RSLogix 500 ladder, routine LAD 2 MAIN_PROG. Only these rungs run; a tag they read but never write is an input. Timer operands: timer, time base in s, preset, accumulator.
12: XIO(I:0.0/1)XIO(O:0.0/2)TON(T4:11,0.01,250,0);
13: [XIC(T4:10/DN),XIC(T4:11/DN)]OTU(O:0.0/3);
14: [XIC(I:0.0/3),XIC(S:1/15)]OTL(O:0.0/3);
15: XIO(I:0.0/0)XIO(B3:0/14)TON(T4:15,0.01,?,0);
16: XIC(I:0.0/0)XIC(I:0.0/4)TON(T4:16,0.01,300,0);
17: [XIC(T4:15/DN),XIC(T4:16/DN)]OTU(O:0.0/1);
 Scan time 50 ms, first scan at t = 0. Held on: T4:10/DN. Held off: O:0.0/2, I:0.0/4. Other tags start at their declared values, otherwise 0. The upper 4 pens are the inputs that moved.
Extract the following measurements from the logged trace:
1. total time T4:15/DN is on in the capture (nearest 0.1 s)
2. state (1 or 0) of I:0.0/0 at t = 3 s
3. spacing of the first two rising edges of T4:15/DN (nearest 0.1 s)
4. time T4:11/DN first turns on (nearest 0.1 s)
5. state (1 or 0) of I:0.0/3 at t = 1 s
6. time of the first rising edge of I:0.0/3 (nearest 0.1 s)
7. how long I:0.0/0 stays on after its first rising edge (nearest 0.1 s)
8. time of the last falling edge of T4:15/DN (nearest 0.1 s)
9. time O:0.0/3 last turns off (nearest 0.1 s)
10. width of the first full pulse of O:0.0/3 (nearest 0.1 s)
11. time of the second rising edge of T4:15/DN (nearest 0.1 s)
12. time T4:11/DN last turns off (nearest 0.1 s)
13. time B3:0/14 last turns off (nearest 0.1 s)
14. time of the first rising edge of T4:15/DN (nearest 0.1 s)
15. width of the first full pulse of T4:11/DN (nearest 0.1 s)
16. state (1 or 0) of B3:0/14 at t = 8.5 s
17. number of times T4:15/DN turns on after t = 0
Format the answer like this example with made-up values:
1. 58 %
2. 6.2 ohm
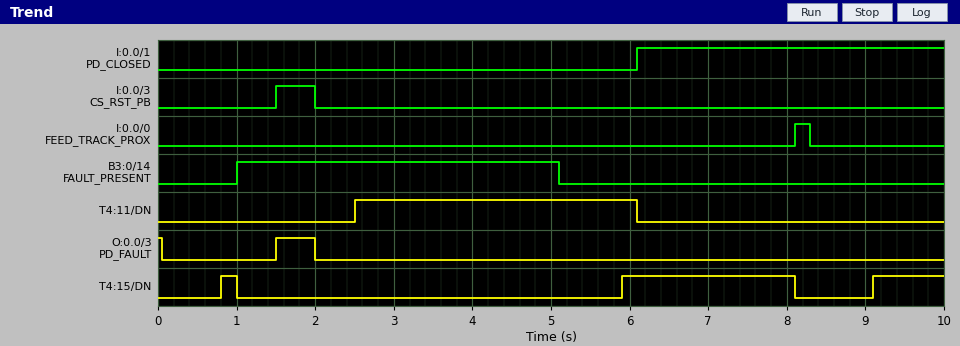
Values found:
1. 3.3 s
2. 0
3. 5.1 s
4. 2.5 s
5. 0
6. 1.5 s
7. 0.2 s
8. 8.1 s
9. 2.0 s
10. 0.5 s
11. 5.9 s
12. 6.1 s
13. 5.1 s
14. 0.8 s
15. 3.6 s
16. 0
17. 3
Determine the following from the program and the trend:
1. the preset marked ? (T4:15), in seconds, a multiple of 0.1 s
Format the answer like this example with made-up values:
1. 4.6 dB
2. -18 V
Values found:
1. 0.8 s
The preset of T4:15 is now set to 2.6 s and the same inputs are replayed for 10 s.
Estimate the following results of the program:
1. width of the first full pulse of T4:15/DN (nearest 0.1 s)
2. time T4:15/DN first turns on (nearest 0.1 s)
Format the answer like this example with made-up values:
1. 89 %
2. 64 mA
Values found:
1. 0.4 s
2. 7.7 s
